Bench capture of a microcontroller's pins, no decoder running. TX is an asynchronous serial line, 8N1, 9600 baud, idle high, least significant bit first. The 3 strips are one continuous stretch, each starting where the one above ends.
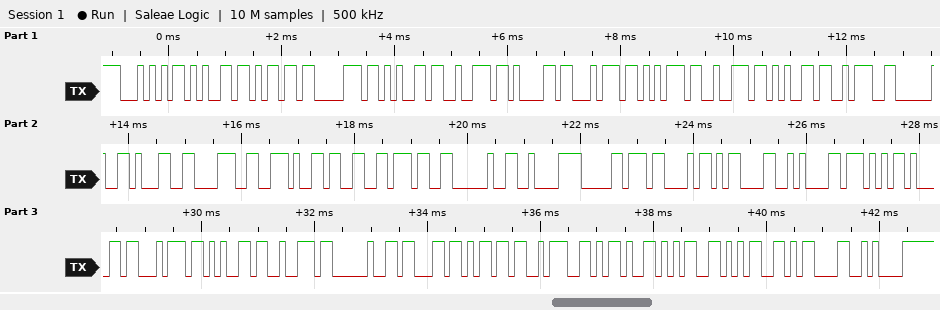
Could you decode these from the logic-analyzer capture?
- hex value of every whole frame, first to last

0x54 0x65 0x6D 0x70 0x65 0x72 0x61 0x74 0x75 0x72 0x65 0x3A 0x20 0x31 0x38 0x2E 0x33 0x37 0x20 0xC2 0xB0 0x43 0x0D 0x0A 0x57 0x61 0x74 0x65 0x72 0x20 0x63 0x6D 0x3A 0x2D 0x35 0x35 0x0D 0x0A
